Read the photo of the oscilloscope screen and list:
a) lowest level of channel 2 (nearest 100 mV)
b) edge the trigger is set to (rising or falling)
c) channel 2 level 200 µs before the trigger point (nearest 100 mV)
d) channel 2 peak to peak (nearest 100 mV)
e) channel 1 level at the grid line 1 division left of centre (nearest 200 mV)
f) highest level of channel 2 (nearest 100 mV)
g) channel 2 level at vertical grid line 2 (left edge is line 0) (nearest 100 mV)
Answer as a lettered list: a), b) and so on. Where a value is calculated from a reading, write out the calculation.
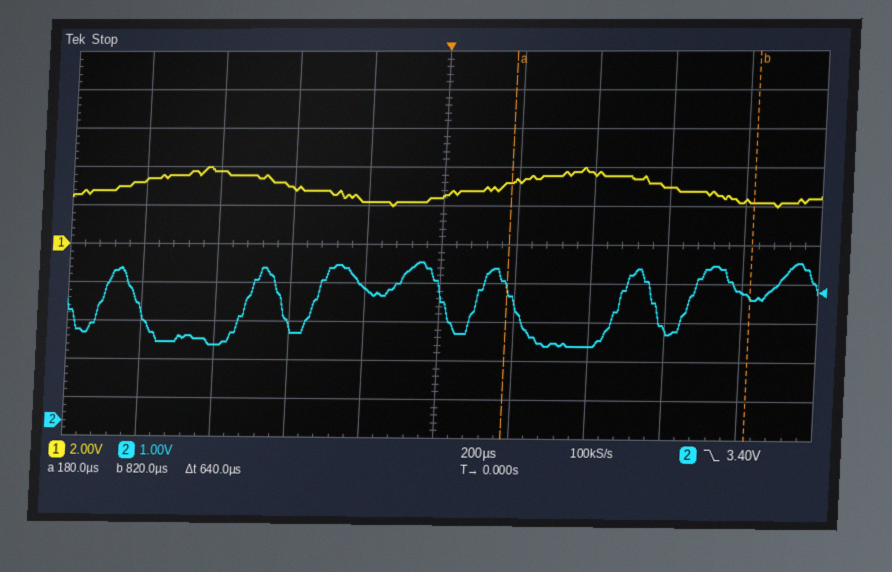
a) 2.0 V
b) falling
c) 3.5 V
d) 4.2 V − (2.0 V) = 2.2 V
e) 2.2 V
f) 4.2 V
g) 2.0 V
